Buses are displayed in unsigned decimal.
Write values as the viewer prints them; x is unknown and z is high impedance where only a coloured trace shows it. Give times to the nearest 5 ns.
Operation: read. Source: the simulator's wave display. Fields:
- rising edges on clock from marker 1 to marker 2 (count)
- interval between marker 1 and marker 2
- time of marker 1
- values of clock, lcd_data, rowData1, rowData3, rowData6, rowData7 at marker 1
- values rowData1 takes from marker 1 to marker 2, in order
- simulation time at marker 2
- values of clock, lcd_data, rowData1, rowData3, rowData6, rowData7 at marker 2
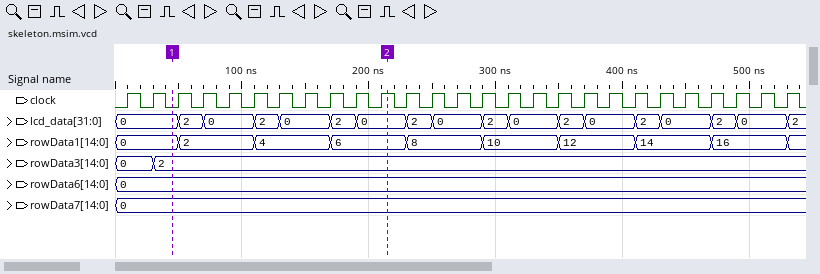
9
170 ns
45 ns
clock=0, lcd_data=0, rowData1=0, rowData3=2, rowData6=0, rowData7=0
0, 2, 4, 6
215 ns
clock=1, lcd_data=0, rowData1=6, rowData3=2, rowData6=0, rowData7=0
